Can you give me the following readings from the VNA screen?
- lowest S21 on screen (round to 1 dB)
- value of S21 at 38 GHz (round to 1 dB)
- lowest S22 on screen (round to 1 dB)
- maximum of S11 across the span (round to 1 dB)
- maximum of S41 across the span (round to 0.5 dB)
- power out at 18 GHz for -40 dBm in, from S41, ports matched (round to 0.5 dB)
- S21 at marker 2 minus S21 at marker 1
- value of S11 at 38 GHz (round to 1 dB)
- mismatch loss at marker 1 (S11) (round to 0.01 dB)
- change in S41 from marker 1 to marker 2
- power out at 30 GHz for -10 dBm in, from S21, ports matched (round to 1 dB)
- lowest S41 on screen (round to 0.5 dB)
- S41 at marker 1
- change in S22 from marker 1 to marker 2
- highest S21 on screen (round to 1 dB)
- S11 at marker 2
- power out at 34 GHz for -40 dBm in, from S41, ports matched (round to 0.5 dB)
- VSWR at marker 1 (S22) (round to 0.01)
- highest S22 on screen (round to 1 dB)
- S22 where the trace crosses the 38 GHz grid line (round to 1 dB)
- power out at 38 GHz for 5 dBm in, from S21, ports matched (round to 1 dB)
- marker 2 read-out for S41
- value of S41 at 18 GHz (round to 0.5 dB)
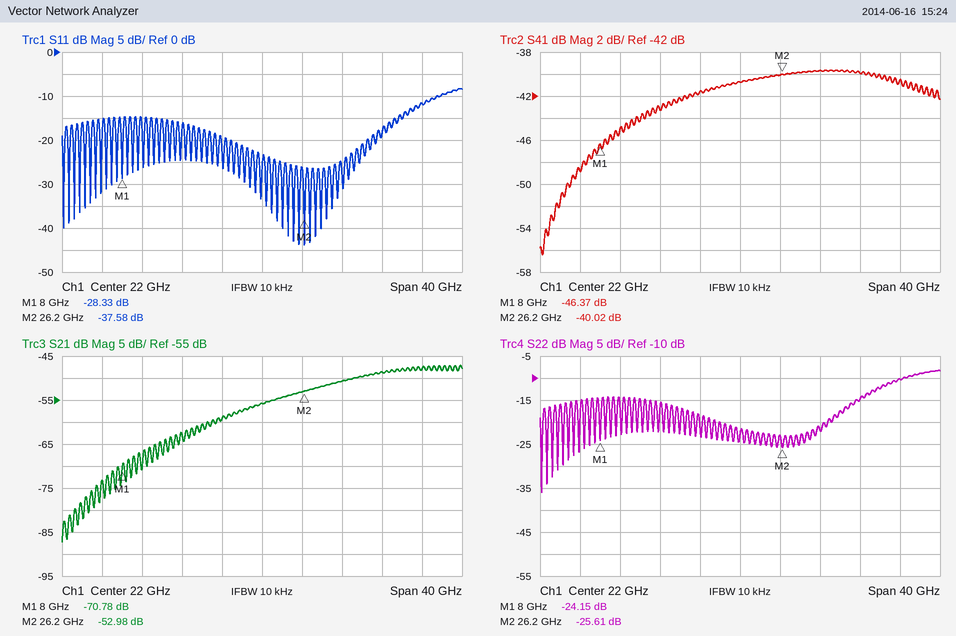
-87 dB
-48 dB
-36 dB
-8 dB
-39.5 dB
-81.5 dBm
17.80 dB
-12 dB
0.01 dB
6.35 dB
-61 dBm
-56.5 dB
-46.37 dB
-1.46 dB
-47 dB
-37.58 dB
-80.0 dBm
1.13
-8 dB
-10 dB
-43 dBm
-40.02 dB
-41.5 dB
